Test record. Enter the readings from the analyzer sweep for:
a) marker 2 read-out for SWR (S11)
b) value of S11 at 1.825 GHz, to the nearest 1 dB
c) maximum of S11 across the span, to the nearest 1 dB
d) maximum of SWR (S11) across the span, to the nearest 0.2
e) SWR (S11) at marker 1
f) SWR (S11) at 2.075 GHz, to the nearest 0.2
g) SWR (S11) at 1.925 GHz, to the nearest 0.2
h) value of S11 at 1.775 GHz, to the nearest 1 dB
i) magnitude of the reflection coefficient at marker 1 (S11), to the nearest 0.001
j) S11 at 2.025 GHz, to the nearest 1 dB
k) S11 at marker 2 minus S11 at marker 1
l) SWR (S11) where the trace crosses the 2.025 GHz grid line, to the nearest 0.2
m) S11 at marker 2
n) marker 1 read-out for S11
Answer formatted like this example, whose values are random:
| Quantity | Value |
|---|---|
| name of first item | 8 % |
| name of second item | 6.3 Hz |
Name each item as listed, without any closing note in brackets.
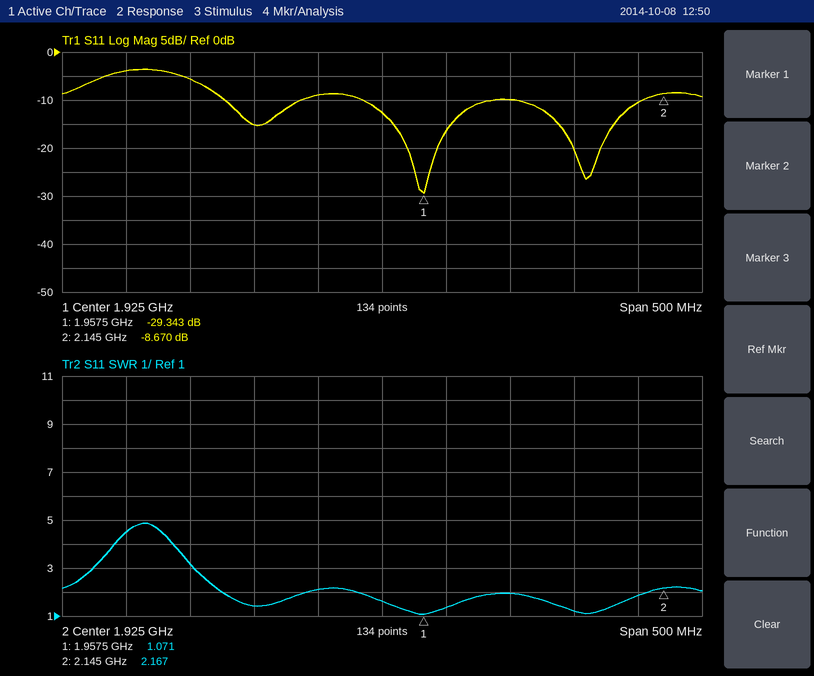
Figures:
| Quantity | Value |
|---|---|
| marker 2 read-out for SWR | 2.167 |
| value of S11 at 1.825 GHz, to the nearest 1 dB | -15 dB |
| maximum of S11 across the span, to the nearest 1 dB | -4 dB |
| maximum of SWR (S11) across the span, to the nearest 0.2 | 4.8 |
| SWR (S11) at marker 1 | 1.071 |
| SWR (S11) at 2.075 GHz, to the nearest 0.2 | 1.2 |
| SWR (S11) at 1.925 GHz, to the nearest 0.2 | 1.6 |
| value of S11 at 1.775 GHz, to the nearest 1 dB | -6 dB |
| magnitude of the reflection coefficient at marker 1 (S11), to the nearest 0.001 | 0.034 |
| S11 at 2.025 GHz, to the nearest 1 dB | -10 dB |
| S11 at marker 2 minus S11 at marker 1 | 20.673 dB |
| SWR (S11) where the trace crosses the 2.025 GHz grid line, to the nearest 0.2 | 2.0 |
| S11 at marker 2 | -8.670 dB |
| marker 1 read-out for S11 | -29.343 dB |
